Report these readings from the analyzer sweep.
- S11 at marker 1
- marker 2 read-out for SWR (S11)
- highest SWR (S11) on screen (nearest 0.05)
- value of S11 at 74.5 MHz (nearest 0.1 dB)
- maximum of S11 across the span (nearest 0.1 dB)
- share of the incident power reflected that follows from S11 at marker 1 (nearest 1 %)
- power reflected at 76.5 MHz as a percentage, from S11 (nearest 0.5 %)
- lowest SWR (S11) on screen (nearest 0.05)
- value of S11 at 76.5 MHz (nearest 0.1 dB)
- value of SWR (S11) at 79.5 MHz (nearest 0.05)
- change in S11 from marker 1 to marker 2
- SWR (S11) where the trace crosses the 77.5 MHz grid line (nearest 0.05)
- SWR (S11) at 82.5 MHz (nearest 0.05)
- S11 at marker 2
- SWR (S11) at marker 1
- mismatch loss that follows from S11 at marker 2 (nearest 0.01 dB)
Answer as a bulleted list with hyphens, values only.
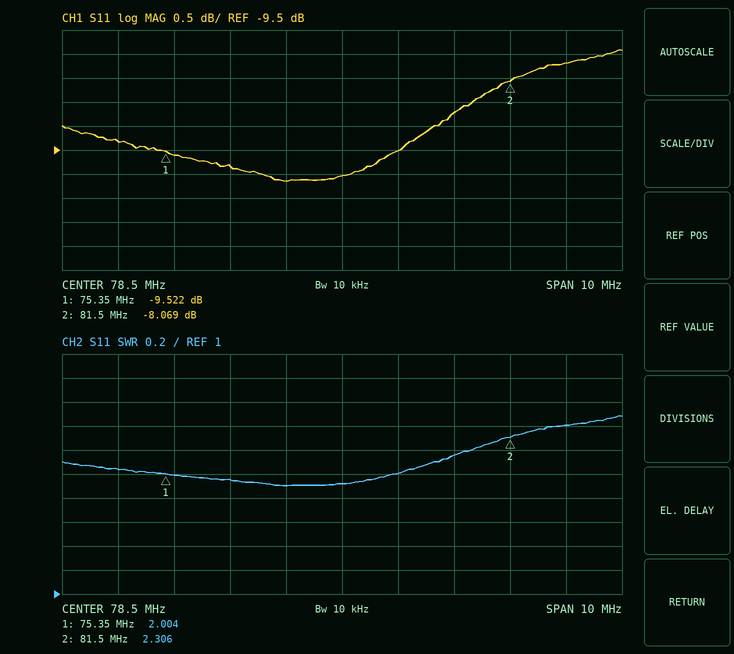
- -9.522 dB
- 2.306
- 2.50
- -9.3 dB
- -7.4 dB
- 11 %
- 10.5 %
- 1.90
- -9.8 dB
- 2.00
- 1.453 dB
- 1.90
- 2.40
- -8.069 dB
- 2.004
- 0.74 dB
